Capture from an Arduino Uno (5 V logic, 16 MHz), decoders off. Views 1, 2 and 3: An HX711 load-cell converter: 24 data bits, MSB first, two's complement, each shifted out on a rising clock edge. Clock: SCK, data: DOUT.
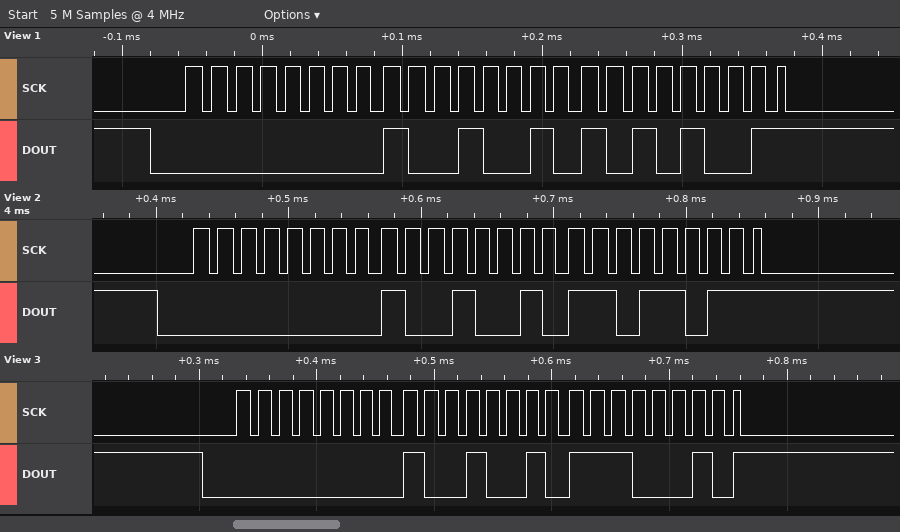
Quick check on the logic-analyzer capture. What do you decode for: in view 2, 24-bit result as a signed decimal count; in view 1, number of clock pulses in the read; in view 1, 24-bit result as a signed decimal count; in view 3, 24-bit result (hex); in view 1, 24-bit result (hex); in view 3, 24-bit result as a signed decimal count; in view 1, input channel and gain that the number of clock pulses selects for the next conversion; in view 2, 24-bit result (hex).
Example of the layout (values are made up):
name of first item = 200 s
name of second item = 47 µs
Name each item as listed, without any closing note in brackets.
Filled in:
in view 2, 24-bit result as a signed decimal count = 37595
in view 1, number of clock pulses in the read = 25
in view 1, 24-bit result as a signed decimal count = 37545
in view 3, 24-bit result = 0x0092E2
in view 1, 24-bit result = 0x0092A9
in view 3, 24-bit result as a signed decimal count = 37602
in view 1, input channel and gain that the number of clock pulses selects for the next conversion = channel A, gain 128
in view 2, 24-bit result = 0x0092DB
